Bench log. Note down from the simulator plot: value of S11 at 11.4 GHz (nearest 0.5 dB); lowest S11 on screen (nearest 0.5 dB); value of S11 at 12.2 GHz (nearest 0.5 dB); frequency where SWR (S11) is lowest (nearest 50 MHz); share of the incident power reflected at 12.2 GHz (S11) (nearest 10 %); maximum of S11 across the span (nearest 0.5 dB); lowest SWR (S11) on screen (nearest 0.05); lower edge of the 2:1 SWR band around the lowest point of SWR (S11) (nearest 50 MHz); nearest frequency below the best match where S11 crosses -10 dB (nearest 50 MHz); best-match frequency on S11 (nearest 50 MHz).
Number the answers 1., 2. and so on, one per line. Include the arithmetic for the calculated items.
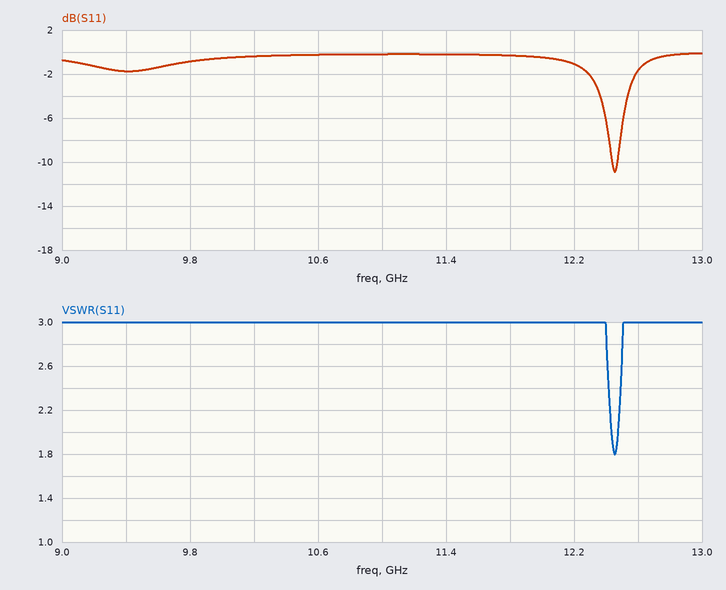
1. 0.0 dB
2. -11.0 dB
3. -1.0 dB
4. 12.45 GHz
5. 10^(-1/10) ≈ 79.4 %, so 80 % to the nearest 10 %
6. 0.0 dB
7. 1.80
8. 12.45 GHz
9. 12.45 GHz
10. 12.45 GHz
